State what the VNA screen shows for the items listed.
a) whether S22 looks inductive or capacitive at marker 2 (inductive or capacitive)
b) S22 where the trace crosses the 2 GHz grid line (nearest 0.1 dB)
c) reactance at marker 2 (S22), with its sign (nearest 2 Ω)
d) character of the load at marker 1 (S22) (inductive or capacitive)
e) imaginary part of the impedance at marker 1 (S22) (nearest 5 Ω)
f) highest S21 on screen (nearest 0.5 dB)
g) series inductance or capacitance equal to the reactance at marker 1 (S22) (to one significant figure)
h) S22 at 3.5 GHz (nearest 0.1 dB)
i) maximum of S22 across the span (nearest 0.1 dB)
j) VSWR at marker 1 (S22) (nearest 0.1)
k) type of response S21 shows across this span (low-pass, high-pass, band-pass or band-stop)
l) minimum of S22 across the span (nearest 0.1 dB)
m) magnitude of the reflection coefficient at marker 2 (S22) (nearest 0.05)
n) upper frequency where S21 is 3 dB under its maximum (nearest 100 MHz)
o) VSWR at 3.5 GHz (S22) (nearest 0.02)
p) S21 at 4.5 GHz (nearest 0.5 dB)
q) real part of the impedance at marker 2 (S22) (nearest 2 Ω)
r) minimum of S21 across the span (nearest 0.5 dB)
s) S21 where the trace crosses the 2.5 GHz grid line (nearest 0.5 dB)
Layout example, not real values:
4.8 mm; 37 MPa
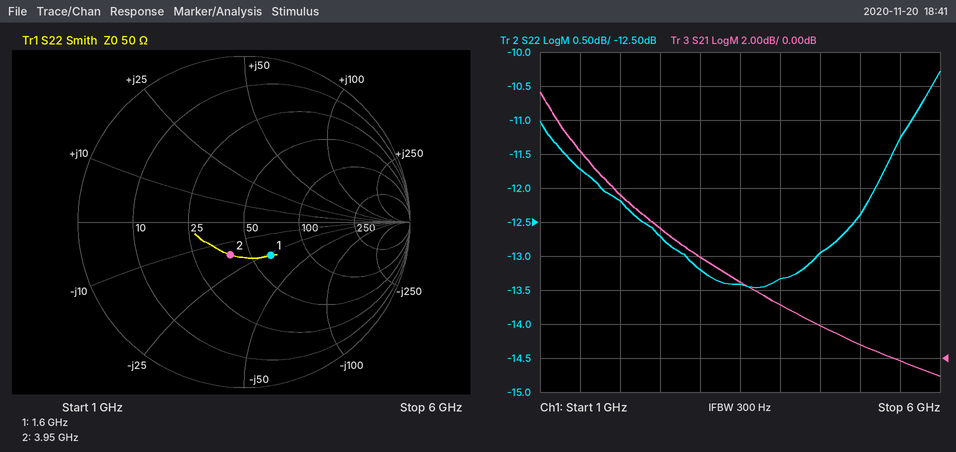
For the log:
capacitive; -12.2 dB; -16 Ω; capacitive; -25 Ω; 15.5 dB; 4 pF; -13.4 dB; -10.3 dB; 1.7; low-pass; -13.5 dB; 0.20; 1.4 GHz; 1.54; 2.0 dB; 40 Ω; -1.0 dB; 7.5 dB
